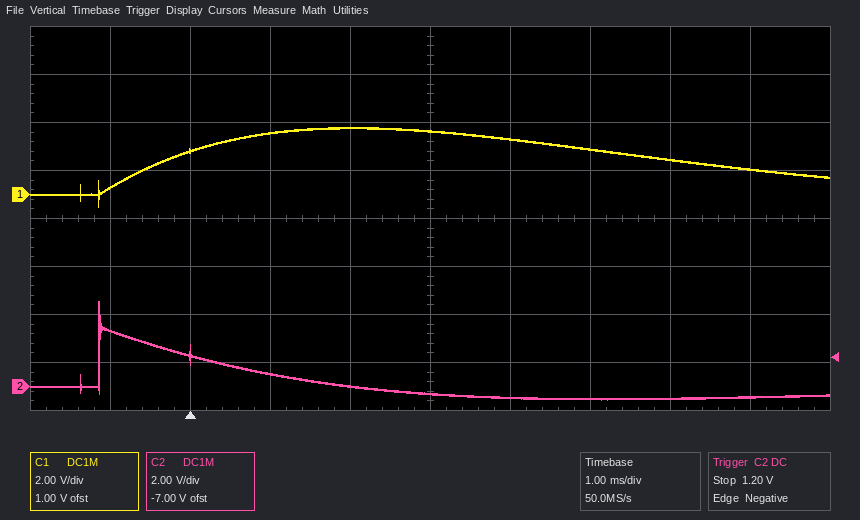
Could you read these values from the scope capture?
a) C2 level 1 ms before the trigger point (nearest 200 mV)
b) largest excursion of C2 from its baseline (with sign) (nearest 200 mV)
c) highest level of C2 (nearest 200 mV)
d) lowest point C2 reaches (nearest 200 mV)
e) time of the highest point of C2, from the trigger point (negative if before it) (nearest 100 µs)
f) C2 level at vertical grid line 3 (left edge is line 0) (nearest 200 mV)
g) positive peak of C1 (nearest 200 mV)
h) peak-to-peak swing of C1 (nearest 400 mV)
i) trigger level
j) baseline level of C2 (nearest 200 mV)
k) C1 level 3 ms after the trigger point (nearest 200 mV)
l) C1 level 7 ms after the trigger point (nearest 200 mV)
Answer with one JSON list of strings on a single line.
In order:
["2.4 V", "+4.0 V", "3.6 V", "-600 mV", "-1.1 ms", "600 mV", "2.8 V", "3.2 V", "1.20 V", "-400 mV", "2.6 V", "1.0 V"]
